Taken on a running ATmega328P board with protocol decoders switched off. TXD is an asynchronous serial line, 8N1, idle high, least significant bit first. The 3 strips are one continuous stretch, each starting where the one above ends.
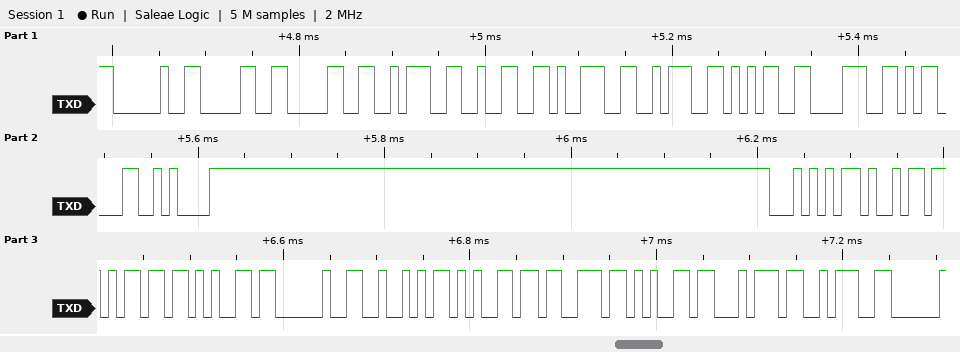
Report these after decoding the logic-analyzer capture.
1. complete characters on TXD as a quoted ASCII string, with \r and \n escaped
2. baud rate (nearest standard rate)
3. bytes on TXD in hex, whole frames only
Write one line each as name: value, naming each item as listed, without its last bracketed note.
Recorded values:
complete characters on TXD as a quoted ASCII string, with \r and \n escaped: " 00:29:58\r\nTime Reset:"
baud rate: 115200 baud
bytes on TXD in hex, whole frames only: 20 30 30 3A 32 39 3A 35 38 0D 0A 54 69 6D 65 20 52 65 73 65 74 3A
